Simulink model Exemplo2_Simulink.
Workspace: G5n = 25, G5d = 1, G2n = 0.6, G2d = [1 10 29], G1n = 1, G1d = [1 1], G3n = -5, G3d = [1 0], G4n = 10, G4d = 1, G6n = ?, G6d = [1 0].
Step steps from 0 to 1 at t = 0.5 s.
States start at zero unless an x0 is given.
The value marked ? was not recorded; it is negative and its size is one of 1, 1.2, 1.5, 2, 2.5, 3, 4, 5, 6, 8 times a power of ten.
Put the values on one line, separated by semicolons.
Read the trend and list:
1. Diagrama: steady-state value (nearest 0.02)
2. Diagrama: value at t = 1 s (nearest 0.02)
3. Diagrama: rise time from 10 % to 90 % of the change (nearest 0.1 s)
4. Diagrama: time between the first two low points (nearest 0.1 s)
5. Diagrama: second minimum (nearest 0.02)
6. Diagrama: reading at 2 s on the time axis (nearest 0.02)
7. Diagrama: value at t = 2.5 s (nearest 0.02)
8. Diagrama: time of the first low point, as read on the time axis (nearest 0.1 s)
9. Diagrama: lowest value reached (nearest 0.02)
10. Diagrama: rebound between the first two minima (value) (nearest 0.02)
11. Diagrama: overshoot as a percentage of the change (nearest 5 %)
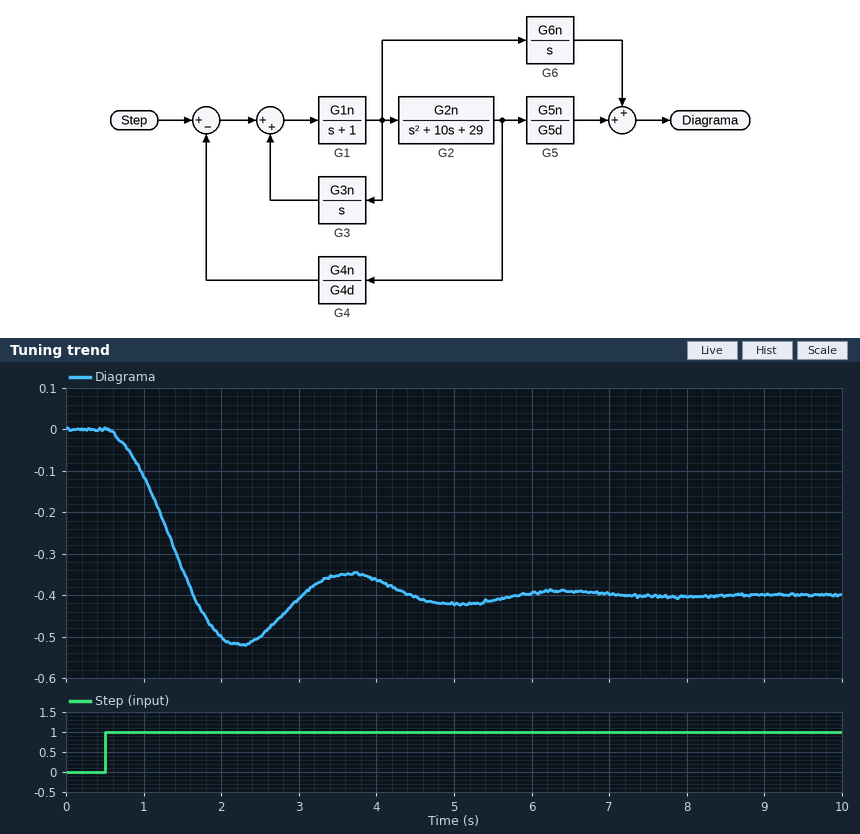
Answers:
-0.40; -0.12; 0.8 s; 2.8 s; -0.42; -0.50; -0.50; 2.2 s; -0.52; -0.34; 30 %
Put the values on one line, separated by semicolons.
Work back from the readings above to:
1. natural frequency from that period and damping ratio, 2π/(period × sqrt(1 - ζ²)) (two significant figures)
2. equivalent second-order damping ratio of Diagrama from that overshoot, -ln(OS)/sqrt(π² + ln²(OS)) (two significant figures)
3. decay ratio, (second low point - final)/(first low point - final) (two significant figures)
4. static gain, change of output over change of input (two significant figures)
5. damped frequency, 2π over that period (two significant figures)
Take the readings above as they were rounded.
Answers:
2.4 rad/s; 0.36; 0.17; -0.40; 2.2 rad/s
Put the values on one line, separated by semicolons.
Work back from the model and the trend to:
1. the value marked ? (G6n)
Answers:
-2
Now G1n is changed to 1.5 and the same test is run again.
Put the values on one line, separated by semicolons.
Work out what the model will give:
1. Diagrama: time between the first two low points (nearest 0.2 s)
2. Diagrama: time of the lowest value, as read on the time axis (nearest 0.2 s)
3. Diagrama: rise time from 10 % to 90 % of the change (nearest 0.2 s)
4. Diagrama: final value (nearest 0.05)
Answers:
2.2 s; 2.0 s; 0.6 s; -0.40
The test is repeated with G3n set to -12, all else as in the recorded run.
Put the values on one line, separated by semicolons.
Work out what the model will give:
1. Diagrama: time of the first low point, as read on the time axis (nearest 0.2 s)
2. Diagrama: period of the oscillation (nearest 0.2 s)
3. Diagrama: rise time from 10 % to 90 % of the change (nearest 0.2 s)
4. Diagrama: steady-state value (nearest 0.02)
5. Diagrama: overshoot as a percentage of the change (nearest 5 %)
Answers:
1.6 s; 1.8 s; 0.6 s; -0.16; 25 %
